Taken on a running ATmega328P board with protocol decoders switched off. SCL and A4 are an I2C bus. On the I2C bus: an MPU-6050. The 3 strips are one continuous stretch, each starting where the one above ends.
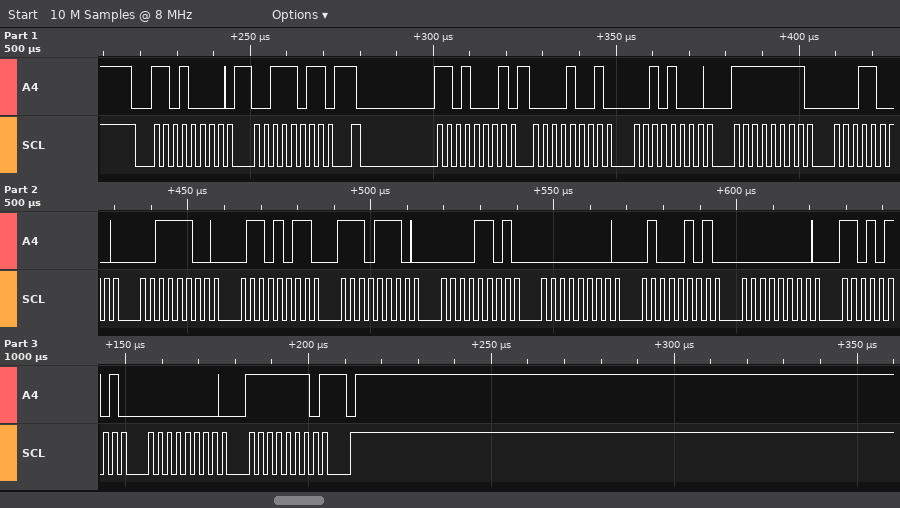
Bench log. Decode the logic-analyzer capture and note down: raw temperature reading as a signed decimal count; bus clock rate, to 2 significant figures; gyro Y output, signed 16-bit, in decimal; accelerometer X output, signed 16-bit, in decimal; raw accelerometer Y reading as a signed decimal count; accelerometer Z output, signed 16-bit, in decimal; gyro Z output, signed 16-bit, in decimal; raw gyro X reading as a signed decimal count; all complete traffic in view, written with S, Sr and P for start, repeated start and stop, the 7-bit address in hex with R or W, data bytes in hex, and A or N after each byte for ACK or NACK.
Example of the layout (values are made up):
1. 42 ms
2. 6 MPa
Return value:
1. -4595
2. 400 kHz
3. 213
4. 2344
5. -232
6. 15467
7. 254
8. 69
9. S 68W A 3B A Sr 68R A 09 A 28 A FF A 18 A 3C A 6B A EE A 0D A 00 A 45 A 00 A D5 A 00 A FE N P
